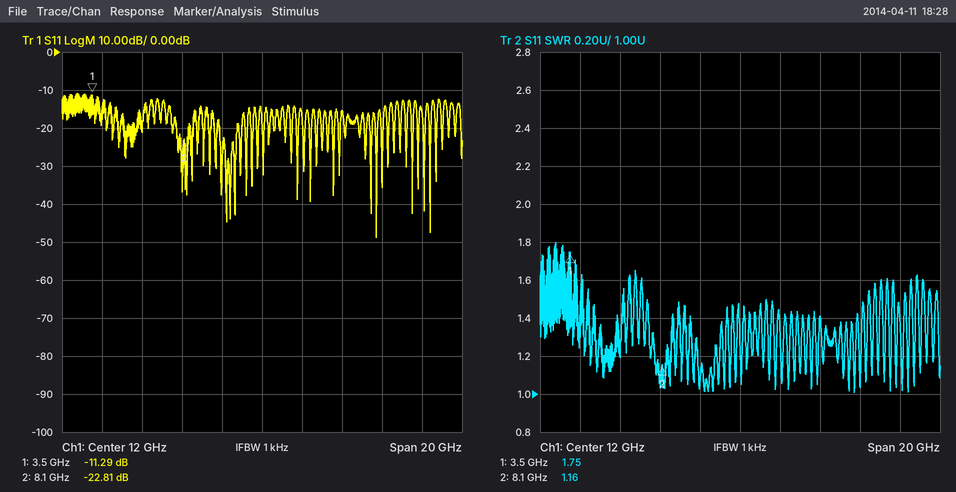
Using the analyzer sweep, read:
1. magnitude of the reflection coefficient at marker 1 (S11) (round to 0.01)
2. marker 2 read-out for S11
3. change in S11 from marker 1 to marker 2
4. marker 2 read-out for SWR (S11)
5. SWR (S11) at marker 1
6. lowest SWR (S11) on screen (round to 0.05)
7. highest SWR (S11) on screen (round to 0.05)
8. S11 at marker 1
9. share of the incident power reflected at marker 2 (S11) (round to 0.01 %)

0.27
-22.81 dB
-11.52 dB
1.16
1.75
1.00
1.80
-11.29 dB
0.52 %
